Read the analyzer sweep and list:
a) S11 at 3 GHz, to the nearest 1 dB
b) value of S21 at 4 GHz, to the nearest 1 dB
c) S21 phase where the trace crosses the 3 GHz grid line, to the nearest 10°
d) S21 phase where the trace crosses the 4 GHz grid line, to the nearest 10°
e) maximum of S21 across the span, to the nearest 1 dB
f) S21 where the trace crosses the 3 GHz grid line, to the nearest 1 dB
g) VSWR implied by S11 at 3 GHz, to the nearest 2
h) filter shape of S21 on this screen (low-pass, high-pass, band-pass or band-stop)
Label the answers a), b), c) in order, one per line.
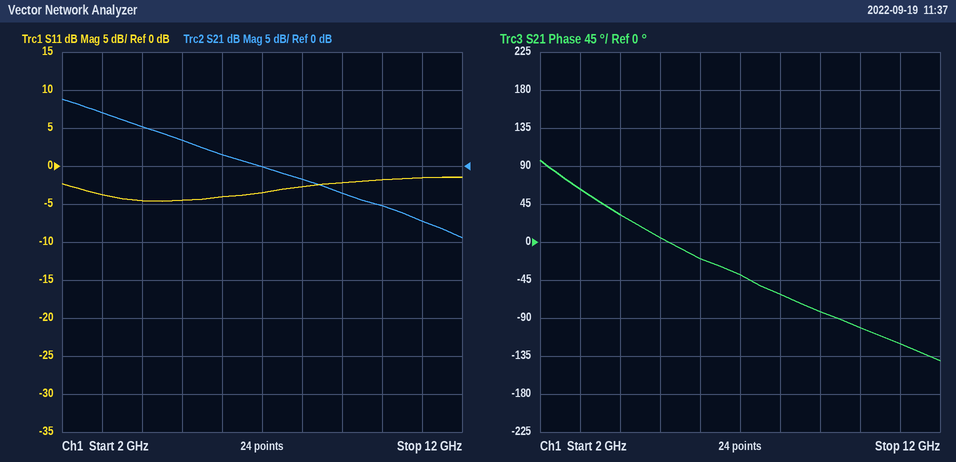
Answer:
a) -4 dB
b) 5 dB
c) 60°
d) 30°
e) 9 dB
f) 7 dB
g) 4
h) low-pass
